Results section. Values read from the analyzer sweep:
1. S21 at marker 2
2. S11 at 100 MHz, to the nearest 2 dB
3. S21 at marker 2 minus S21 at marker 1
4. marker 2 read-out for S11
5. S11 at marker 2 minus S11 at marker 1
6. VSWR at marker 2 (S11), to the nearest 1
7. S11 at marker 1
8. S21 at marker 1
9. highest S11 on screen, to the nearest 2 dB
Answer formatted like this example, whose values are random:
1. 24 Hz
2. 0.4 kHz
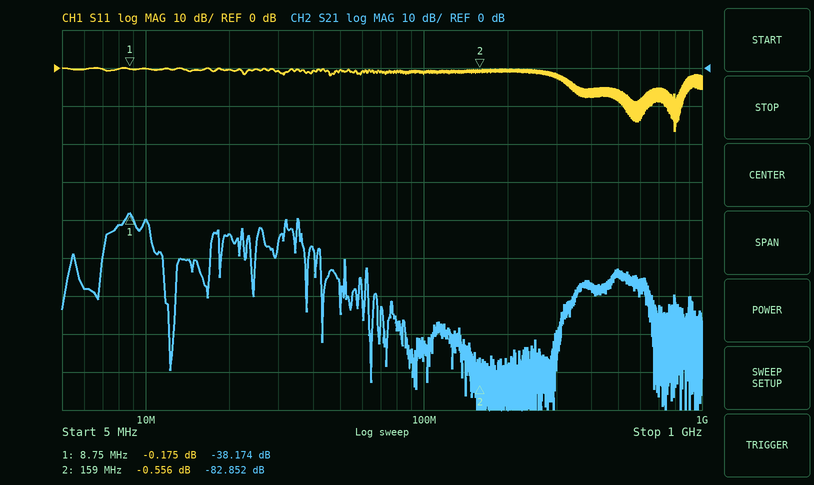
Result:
1. -82.852 dB
2. -2 dB
3. -44.678 dB
4. -0.556 dB
5. -0.381 dB
6. 31
7. -0.175 dB
8. -38.174 dB
9. 0 dB
